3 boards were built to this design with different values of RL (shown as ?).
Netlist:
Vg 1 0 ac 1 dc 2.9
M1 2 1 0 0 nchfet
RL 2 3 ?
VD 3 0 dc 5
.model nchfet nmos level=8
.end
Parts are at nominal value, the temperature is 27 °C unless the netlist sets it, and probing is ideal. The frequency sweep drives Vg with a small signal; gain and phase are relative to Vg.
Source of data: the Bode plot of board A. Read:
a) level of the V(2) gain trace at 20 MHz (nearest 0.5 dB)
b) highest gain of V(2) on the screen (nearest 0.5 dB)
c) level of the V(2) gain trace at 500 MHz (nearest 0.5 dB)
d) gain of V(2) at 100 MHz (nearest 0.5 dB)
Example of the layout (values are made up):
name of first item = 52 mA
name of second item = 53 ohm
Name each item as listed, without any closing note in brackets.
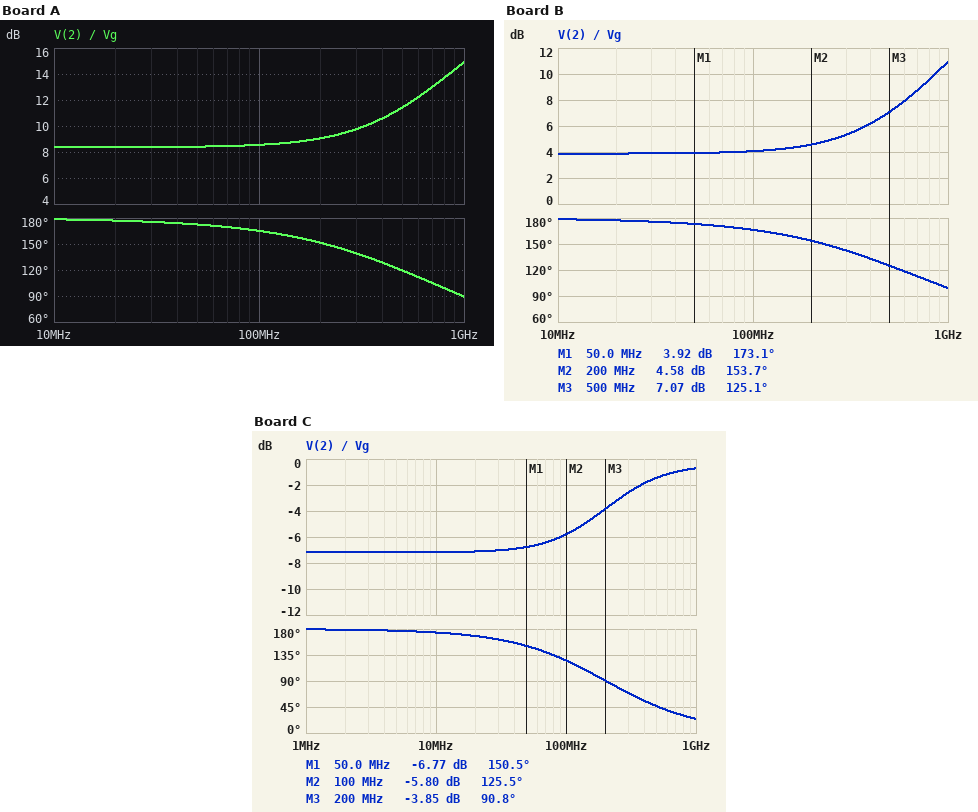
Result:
level of the V(2) gain trace at 20 MHz = 8.5 dB
highest gain of V(2) on the screen = 15.0 dB
level of the V(2) gain trace at 500 MHz = 11.5 dB
gain of V(2) at 100 MHz = 8.5 dB
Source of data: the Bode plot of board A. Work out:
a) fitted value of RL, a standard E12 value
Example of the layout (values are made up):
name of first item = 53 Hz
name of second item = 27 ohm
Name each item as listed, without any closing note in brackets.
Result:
fitted value of RL, a standard E12 value = 56 kΩ
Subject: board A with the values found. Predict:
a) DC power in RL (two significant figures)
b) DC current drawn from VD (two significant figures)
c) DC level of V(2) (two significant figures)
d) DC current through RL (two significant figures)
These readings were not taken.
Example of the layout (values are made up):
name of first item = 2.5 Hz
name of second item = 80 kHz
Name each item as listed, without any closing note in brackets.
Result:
DC power in RL = 51 µW
DC current drawn from VD = 30 µA
DC level of V(2) = 3.3 V
DC current through RL = 30 µA
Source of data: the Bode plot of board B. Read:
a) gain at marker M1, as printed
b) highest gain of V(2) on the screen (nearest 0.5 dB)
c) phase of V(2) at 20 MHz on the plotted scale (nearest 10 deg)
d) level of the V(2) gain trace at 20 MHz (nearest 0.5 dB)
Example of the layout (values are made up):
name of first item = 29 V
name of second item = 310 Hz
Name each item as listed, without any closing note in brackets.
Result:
gain at marker M1, as printed = 3.92 dB
highest gain of V(2) on the screen = 11.0 dB
phase of V(2) at 20 MHz on the plotted scale = 180 deg
level of the V(2) gain trace at 20 MHz = 4.0 dB
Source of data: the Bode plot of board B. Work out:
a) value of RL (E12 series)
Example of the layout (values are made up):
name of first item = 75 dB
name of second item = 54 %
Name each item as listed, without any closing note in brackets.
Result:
value of RL = 33 kΩ
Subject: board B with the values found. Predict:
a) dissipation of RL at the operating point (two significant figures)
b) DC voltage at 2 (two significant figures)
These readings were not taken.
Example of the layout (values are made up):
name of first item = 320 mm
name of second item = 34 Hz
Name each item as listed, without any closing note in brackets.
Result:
dissipation of RL at the operating point = 31 µW
DC voltage at 2 = 4.0 V
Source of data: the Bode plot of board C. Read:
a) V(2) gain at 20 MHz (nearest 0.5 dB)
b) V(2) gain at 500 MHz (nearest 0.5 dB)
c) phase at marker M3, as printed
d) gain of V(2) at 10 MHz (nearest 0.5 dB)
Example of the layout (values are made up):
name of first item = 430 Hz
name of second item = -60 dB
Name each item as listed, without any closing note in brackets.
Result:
V(2) gain at 20 MHz = -7.0 dB
V(2) gain at 500 MHz = -1.5 dB
phase at marker M3, as printed = 90.8 deg
gain of V(2) at 10 MHz = -7.0 dB
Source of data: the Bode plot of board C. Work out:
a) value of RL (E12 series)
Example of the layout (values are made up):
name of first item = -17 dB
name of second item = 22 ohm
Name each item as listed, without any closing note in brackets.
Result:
value of RL = 220 kΩ
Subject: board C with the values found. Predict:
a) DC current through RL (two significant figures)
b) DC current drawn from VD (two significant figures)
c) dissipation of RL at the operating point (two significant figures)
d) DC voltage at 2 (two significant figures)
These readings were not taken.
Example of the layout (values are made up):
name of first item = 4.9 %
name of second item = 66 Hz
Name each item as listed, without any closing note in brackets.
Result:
DC current through RL = 21 µA
DC current drawn from VD = 21 µA
dissipation of RL at the operating point = 100 µW
DC voltage at 2 = 290 mV
